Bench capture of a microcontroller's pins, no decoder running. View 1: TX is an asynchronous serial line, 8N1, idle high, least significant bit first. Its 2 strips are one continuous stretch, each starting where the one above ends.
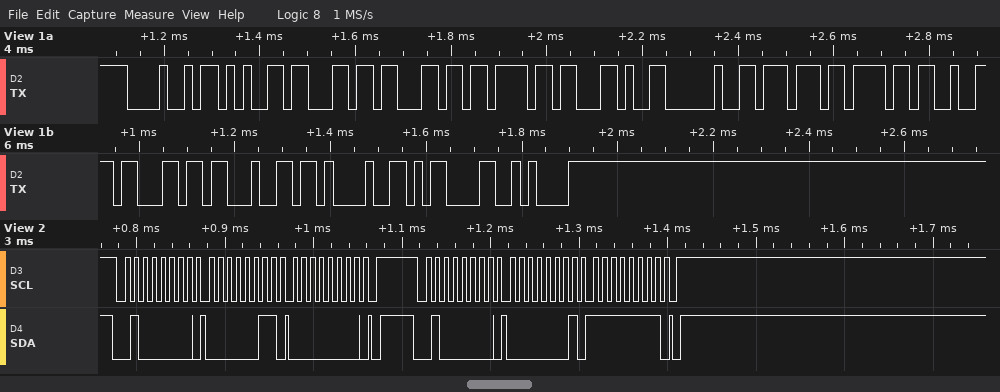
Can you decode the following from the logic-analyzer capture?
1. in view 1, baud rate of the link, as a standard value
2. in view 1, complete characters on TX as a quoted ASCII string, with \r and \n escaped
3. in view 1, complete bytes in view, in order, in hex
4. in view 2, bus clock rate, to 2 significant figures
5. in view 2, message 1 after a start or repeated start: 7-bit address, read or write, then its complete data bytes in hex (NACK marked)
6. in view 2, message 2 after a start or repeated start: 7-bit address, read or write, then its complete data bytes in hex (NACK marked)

57600 baud
"Hello, world!\r\n"
48 65 6C 6C 6F 2C 20 77 6F 72 6C 64 21 0D 0A
100 kHz
0x20 write: 03 00
0x20 write: 01 FF
